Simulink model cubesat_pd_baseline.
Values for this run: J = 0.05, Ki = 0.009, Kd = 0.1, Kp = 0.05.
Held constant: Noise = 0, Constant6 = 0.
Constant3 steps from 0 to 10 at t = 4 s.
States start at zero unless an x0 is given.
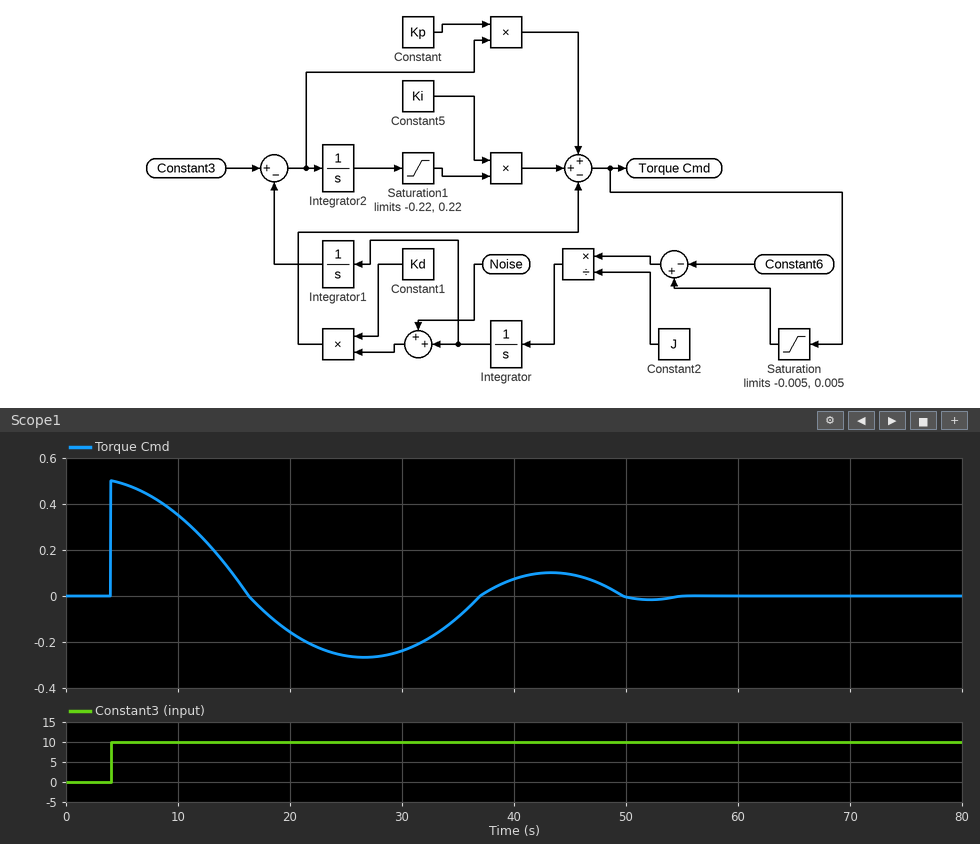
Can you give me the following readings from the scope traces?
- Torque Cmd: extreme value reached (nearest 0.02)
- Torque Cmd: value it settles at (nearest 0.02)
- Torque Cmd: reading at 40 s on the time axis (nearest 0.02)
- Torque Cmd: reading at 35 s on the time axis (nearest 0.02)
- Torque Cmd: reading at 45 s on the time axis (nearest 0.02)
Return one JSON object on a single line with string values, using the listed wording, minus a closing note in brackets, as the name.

{"Torque Cmd: extreme value reached": "0.50", "Torque Cmd: value it settles at": "0.00", "Torque Cmd: reading at 40 s on the time axis": "0.08", "Torque Cmd: reading at 35 s on the time axis": "-0.10", "Torque Cmd: reading at 45 s on the time axis": "0.10"}
